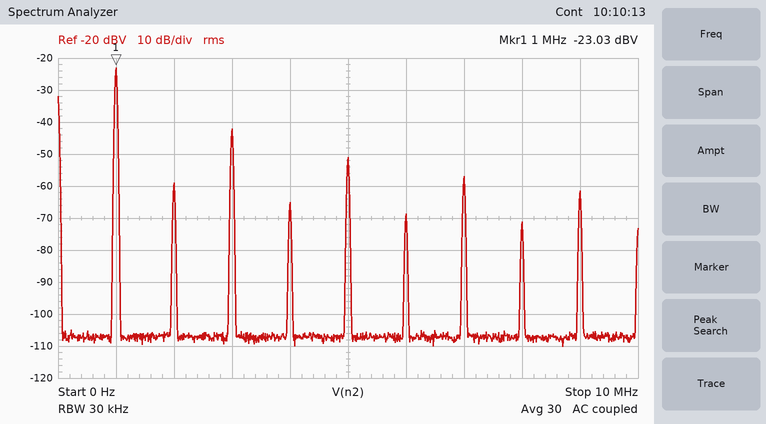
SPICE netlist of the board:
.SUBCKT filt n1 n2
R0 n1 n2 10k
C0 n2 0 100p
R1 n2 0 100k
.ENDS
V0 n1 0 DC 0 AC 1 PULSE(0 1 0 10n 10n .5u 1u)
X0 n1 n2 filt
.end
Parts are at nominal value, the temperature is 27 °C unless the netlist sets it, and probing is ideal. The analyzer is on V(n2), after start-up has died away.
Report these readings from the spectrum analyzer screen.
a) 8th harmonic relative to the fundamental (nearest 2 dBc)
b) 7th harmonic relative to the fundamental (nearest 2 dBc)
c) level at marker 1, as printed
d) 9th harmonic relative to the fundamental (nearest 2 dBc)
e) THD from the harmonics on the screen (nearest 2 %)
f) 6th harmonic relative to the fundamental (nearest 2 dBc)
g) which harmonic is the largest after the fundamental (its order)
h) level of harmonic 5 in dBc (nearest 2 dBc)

-48 dBc
-34 dBc
-23.03 dBV
-38 dBc
12 %
-46 dBc
3
-28 dBc
